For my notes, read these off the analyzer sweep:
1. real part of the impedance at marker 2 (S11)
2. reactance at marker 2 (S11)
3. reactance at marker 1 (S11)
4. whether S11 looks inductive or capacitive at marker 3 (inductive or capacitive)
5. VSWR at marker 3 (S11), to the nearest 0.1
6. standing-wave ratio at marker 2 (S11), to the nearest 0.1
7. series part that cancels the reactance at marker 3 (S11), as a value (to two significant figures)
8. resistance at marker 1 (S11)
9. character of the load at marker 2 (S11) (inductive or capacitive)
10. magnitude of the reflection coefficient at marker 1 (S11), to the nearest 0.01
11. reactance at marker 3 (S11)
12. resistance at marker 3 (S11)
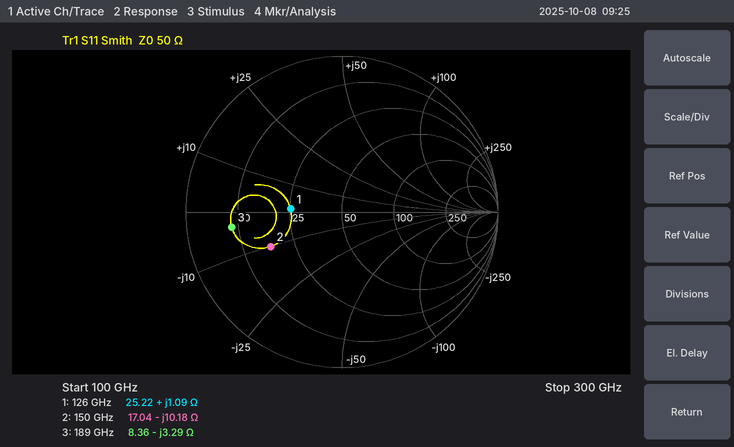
17.04 Ω
-10.18 Ω
+1.09 Ω
capacitive
6.0
3.1
2.8 pH
25.22 Ω
capacitive
0.33
-3.29 Ω
8.36 Ω
